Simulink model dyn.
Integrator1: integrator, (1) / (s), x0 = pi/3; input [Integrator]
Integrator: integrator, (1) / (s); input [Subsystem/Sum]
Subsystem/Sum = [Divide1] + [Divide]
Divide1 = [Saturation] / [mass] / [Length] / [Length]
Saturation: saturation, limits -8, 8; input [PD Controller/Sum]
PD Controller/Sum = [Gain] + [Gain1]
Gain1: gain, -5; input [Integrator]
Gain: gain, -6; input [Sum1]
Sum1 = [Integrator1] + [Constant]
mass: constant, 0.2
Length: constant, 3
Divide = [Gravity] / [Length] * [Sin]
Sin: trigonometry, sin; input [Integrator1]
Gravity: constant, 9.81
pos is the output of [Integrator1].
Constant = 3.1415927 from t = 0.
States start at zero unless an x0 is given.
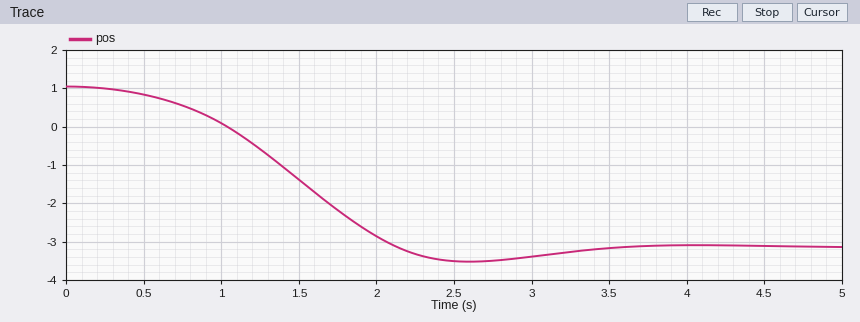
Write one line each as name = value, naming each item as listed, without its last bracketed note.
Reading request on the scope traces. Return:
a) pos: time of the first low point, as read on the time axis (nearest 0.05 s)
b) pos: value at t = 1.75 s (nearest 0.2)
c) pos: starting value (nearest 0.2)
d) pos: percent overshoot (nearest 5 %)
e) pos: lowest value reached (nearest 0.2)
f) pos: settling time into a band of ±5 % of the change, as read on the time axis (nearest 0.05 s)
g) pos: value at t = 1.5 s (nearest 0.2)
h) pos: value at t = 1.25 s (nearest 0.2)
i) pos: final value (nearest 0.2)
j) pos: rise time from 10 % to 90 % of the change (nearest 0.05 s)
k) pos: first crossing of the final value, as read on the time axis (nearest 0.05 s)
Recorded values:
pos: time of the first low point, as read on the time axis = 2.60 s
pos: value at t = 1.75 s = -2.2
pos: starting value = 1.0
pos: percent overshoot = 10 %
pos: lowest value reached = -3.6
pos: settling time into a band of ±5 % of the change, as read on the time axis = 3.10 s
pos: value at t = 1.5 s = -1.4
pos: value at t = 1.25 s = -0.6
pos: final value = -3.2
pos: rise time from 10 % to 90 % of the change = 1.25 s
pos: first crossing of the final value, as read on the time axis = 2.15 s
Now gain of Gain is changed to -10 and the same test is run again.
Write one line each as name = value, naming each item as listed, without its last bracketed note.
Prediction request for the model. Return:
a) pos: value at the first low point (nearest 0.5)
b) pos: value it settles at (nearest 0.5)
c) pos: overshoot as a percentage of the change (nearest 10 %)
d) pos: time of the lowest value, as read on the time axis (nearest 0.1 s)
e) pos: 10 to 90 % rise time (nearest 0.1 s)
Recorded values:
pos: value at the first low point = -4.0
pos: value it settles at = -3.0
pos: overshoot as a percentage of the change = 20 %
pos: time of the lowest value, as read on the time axis = 2.4 s
pos: 10 to 90 % rise time = 1.1 s
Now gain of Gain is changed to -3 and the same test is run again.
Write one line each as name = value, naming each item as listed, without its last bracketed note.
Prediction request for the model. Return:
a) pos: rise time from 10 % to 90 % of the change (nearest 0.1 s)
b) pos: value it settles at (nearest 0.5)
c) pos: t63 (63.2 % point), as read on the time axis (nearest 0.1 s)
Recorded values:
pos: rise time from 10 % to 90 % of the change = 1.9 s
pos: value it settles at = -3.0
pos: t63 (63.2 % point), as read on the time axis = 2.0 s
